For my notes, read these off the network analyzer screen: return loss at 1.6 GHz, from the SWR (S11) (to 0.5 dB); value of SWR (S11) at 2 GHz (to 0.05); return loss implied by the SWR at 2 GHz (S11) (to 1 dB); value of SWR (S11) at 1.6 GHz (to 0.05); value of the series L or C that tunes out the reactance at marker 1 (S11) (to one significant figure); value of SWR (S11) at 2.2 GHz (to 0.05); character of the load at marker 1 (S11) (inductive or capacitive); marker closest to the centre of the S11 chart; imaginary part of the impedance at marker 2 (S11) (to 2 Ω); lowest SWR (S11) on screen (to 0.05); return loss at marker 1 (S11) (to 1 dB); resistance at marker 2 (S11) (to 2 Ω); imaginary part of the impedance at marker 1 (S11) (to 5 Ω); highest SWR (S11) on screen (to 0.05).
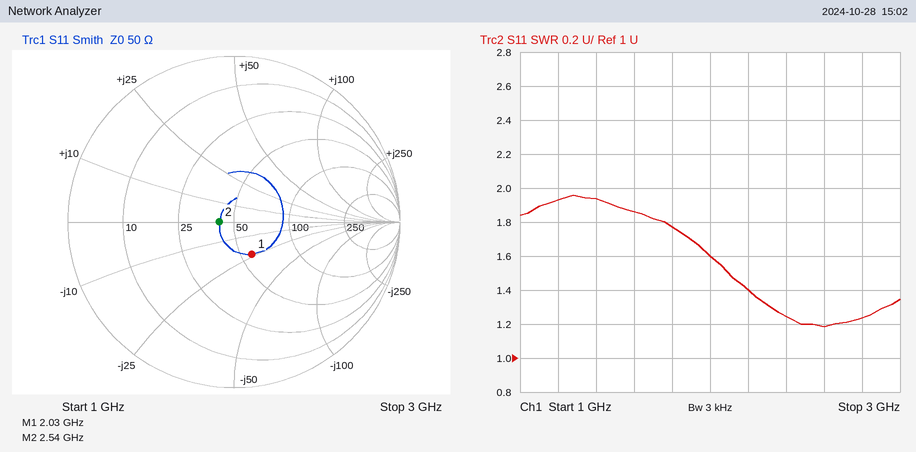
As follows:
10.5 dB
1.60
13 dB
1.85
2 nH
1.40
capacitive
marker 2
0 Ω
1.20
13 dB
42 Ω
-25 Ω
1.95
